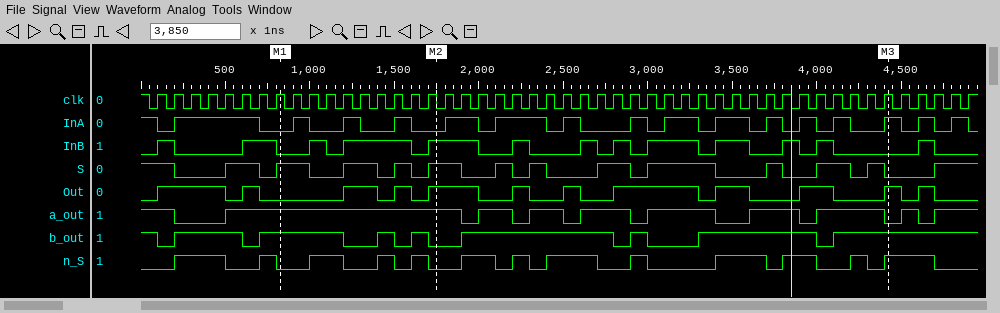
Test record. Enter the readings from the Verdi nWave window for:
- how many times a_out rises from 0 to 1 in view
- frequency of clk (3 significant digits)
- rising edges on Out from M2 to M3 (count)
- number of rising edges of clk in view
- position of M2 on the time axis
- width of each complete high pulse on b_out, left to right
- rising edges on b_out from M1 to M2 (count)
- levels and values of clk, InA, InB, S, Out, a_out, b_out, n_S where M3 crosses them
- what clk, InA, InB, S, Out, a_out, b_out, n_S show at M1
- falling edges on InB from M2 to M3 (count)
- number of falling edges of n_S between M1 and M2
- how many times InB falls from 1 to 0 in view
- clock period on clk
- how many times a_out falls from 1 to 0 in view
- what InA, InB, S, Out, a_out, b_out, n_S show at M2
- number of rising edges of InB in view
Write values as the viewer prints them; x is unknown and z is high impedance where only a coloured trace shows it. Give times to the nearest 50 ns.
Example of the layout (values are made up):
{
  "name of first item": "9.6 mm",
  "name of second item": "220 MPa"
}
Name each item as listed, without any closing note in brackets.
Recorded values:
{
  "how many times a_out rises from 0 to 1 in view": "9",
  "frequency of clk": "10.0 MHz",
  "rising edges on Out from M2 to M3": "6",
  "number of rising edges of clk in view": "49",
  "position of M2 on the time axis": "1750 ns",
  "width of each complete high pulse on b_out, left to right": "400 ns, 500 ns, 100 ns, 100 ns, 900 ns, 100 ns, 700 ns",
  "rising edges on b_out from M1 to M2": "2",
  "levels and values of clk, InA, InB, S, Out, a_out, b_out, n_S where M3 crosses them": "clk=1, InA=1, InB=0, S=0, Out=1, a_out=0, b_out=1, n_S=1",
  "what clk, InA, InB, S, Out, a_out, b_out, n_S show at M1": "clk=1, InA=0, InB=0, S=1, Out=0, a_out=1, b_out=1, n_S=0",
  "falling edges on InB from M2 to M3": "8",
  "number of falling edges of n_S between M1 and M2": "3",
  "how many times InB falls from 1 to 0 in view": "13",
  "clock period on clk": "100 ns",
  "how many times a_out falls from 1 to 0 in view": "9",
  "what InA, InB, S, Out, a_out, b_out, n_S show at M2": "InA=0, InB=1, S=1, Out=1, a_out=1, b_out=0, n_S=0",
  "number of rising edges of InB in view": "13"
}
